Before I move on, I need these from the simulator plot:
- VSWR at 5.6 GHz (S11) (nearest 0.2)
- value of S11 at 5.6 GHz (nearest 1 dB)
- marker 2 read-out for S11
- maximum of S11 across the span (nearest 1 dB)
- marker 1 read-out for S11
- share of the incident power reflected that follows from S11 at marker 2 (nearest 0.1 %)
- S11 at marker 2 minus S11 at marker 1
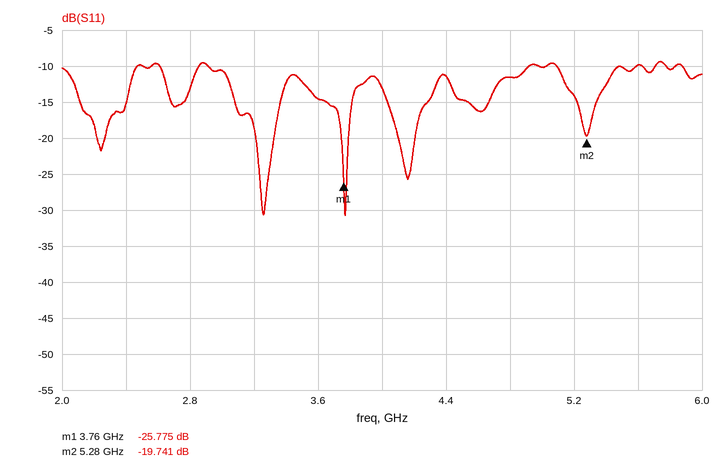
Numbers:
2.0
-10 dB
-19.741 dB
-9 dB
-25.775 dB
1.1 %
6.034 dB
